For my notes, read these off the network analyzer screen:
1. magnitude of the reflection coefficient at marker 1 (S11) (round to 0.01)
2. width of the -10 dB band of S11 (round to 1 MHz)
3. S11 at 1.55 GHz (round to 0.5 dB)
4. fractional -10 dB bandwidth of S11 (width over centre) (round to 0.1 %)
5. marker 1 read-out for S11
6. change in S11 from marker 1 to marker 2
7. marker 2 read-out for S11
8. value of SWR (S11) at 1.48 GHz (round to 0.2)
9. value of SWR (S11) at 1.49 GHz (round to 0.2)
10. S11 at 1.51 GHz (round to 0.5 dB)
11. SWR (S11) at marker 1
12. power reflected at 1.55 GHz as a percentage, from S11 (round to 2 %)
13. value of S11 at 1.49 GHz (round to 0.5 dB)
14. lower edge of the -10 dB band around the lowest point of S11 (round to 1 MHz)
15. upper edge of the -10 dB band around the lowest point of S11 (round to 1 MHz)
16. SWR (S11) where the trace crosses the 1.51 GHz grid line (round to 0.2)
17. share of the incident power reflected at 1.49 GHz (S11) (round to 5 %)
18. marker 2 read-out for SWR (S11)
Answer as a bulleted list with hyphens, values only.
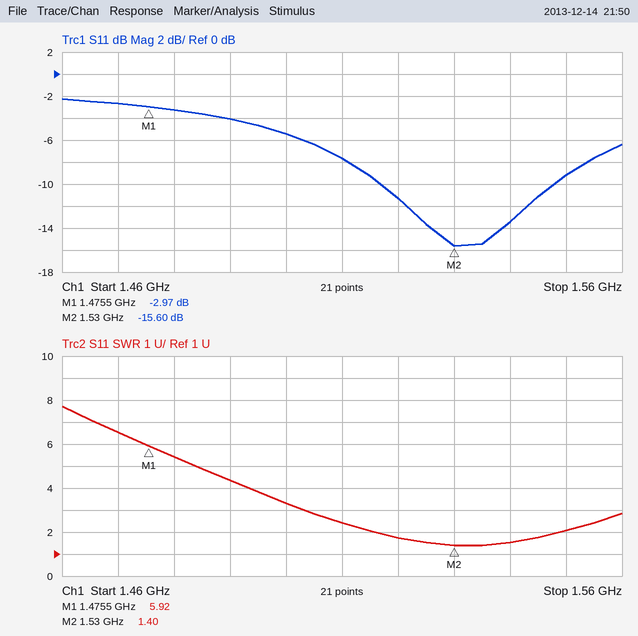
- 0.71
- 31 MHz
- -9.0 dB
- 2.0 %
- -2.97 dB
- -12.63 dB
- -15.60 dB
- 5.4
- 4.4
- -7.5 dB
- 5.92
- 12 %
- -4.0 dB
- 1.517 GHz
- 1.548 GHz
- 2.4
- 40 %
- 1.40
